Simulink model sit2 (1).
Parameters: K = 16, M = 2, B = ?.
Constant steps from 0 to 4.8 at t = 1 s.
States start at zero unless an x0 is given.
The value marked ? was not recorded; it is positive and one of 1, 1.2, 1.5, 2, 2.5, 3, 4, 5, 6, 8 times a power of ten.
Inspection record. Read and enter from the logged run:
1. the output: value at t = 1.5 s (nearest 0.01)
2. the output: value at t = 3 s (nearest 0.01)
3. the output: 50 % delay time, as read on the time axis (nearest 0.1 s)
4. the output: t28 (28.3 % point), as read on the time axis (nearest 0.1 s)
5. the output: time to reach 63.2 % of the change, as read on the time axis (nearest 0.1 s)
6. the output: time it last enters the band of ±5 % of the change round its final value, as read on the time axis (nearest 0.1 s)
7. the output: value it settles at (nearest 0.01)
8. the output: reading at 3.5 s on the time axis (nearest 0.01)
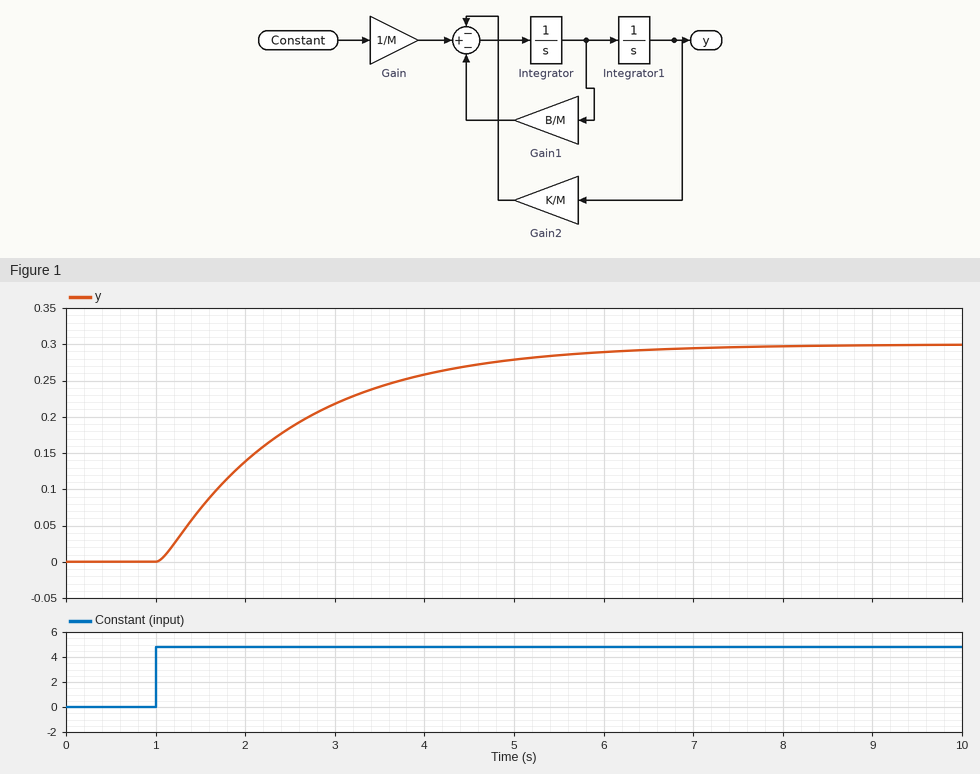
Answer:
0.07
0.22
2.1 s
1.6 s
2.6 s
5.5 s
0.30
0.24
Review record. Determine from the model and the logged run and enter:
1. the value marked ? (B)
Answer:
25
